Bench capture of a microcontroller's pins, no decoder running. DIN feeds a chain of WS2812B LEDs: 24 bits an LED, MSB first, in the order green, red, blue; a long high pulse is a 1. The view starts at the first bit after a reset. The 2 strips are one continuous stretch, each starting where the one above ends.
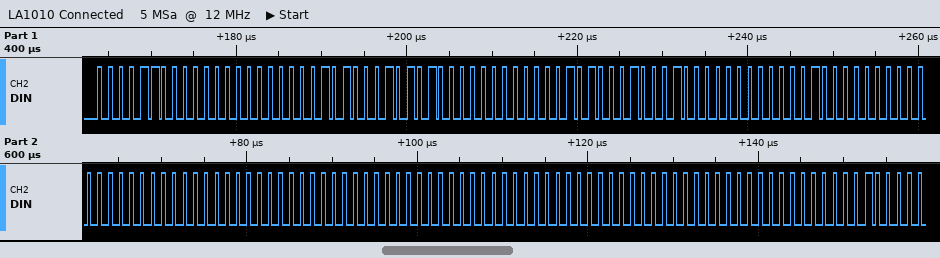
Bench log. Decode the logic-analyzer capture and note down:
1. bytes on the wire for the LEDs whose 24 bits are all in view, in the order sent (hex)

0C 00 05 15 00 0A 22 00 10 00 00 00 00 00 00 00 00 00
